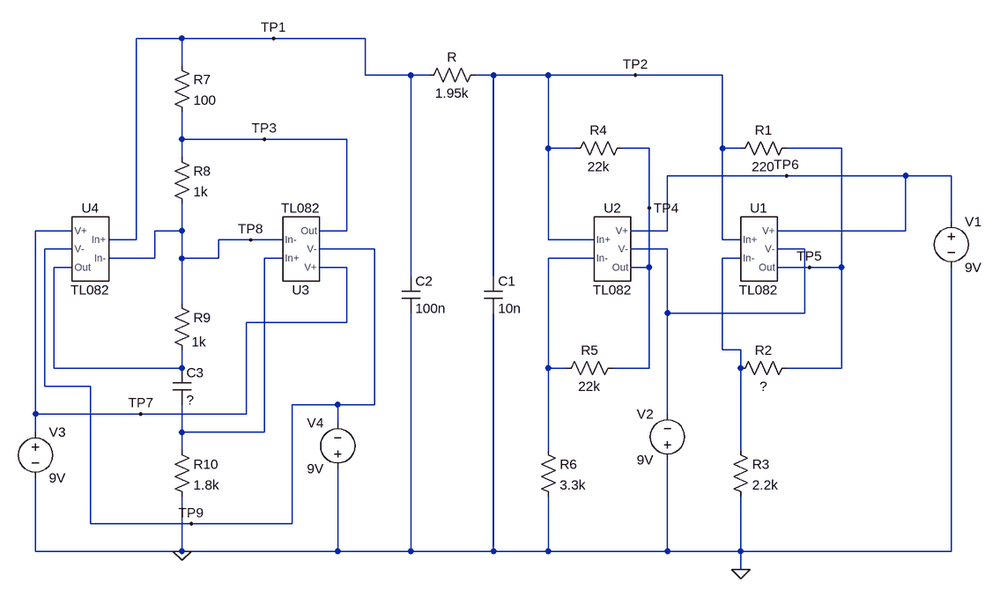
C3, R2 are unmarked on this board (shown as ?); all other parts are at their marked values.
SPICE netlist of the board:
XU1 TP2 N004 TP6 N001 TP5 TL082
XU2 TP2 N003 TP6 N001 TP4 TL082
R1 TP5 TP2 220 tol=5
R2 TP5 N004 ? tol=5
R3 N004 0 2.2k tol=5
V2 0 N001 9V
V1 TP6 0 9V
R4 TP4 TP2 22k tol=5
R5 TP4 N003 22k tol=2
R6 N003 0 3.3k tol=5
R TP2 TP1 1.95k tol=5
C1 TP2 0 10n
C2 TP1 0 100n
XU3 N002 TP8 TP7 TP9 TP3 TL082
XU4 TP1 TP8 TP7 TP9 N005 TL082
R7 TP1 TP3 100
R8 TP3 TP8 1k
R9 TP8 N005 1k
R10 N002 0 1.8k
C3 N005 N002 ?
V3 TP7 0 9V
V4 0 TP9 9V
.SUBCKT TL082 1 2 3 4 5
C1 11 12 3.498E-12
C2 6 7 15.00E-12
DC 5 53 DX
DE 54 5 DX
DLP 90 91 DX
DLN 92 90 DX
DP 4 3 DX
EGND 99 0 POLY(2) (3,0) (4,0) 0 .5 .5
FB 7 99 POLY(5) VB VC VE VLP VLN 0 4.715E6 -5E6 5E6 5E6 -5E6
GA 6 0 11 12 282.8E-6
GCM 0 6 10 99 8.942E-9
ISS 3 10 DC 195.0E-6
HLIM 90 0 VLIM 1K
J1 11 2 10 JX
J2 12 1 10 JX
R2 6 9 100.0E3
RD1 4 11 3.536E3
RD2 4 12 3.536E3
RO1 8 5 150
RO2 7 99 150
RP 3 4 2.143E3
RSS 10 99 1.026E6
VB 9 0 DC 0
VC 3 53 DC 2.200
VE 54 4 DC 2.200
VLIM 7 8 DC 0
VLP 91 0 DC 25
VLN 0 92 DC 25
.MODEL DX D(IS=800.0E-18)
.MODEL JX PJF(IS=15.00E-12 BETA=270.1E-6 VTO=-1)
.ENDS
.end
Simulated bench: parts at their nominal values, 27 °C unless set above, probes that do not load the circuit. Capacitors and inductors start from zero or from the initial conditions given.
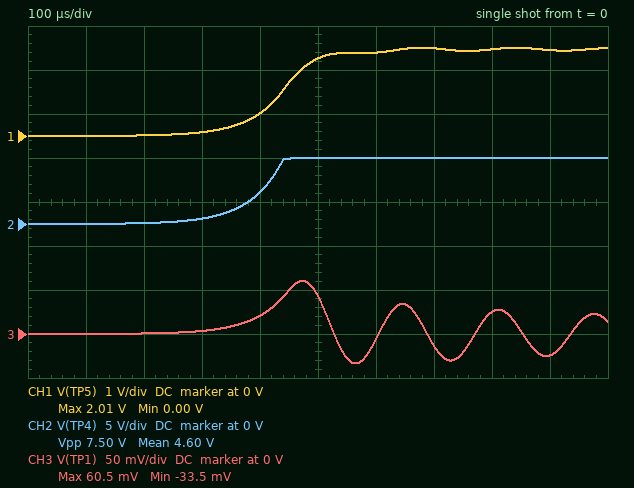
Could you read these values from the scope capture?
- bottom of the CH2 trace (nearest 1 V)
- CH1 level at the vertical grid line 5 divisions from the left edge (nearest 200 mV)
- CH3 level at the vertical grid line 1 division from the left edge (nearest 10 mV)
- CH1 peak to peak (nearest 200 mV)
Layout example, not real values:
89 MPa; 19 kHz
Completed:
0 V; 1.8 V; 0 V; 2.0 V
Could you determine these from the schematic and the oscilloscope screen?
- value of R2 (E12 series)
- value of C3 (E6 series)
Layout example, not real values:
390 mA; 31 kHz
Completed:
180 Ω; 33 nF
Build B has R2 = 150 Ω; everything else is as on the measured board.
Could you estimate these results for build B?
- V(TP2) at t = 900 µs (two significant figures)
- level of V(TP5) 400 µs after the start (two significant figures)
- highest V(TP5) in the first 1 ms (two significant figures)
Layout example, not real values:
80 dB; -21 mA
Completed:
1.4 V; 56 mV; 1.5 V
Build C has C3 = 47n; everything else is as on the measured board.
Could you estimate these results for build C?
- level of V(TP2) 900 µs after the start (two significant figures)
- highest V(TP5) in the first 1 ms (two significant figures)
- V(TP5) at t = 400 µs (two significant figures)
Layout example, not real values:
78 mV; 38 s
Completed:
1.9 V; 2.1 V; 700 mV
